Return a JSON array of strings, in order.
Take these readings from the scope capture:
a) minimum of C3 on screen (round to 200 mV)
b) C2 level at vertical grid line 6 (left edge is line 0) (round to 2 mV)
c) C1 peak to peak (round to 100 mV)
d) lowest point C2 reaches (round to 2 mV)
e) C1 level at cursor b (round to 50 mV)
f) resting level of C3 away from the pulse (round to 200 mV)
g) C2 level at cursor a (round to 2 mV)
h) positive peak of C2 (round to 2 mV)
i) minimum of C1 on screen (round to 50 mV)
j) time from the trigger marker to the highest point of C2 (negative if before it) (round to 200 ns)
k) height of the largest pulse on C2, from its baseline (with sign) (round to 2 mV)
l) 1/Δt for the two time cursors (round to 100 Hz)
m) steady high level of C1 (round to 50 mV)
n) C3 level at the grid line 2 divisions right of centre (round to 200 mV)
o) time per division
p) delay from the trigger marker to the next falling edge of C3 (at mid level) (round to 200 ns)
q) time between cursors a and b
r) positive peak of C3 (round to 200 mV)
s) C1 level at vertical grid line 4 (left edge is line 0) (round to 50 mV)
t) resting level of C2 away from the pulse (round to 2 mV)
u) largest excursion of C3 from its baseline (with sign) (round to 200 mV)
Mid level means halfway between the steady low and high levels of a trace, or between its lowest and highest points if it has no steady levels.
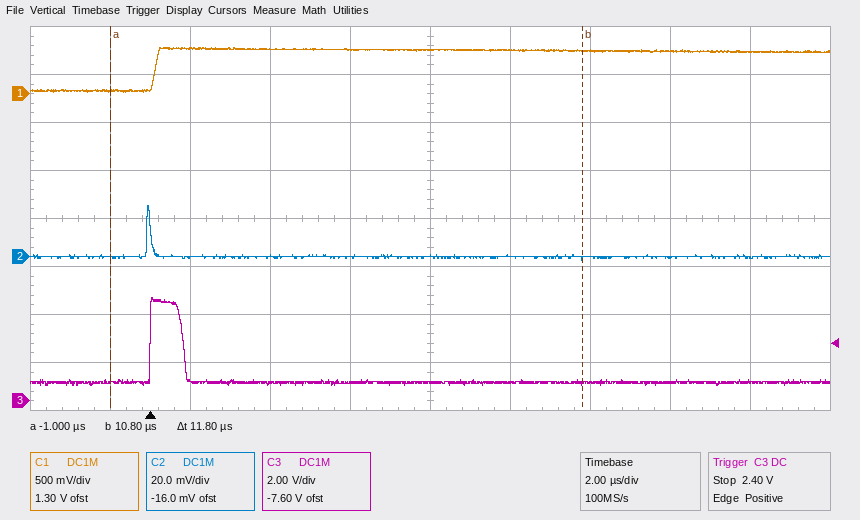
["600 mV", "0 mV", "500 mV", "-2 mV", "450 mV", "800 mV", "0 mV", "22 mV", "0 mV", "0.0 µs", "+22 mV", "84.7 kHz", "450 mV", "800 mV", "2 µs", "800 ns", "11.8 µs", "4.4 V", "450 mV", "0 mV", "+3.6 V"]
